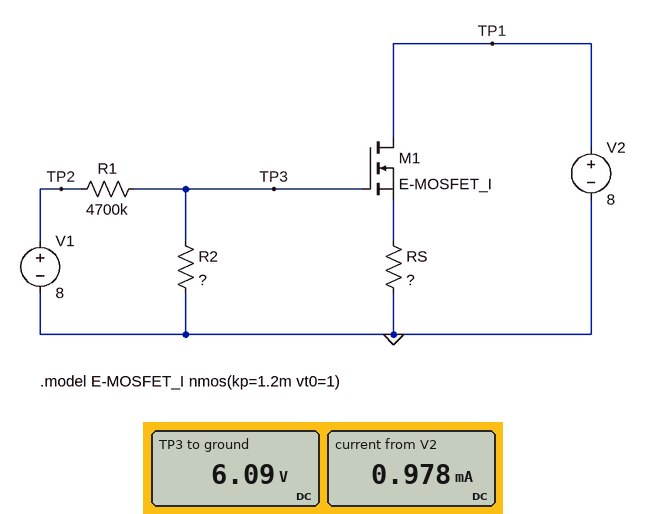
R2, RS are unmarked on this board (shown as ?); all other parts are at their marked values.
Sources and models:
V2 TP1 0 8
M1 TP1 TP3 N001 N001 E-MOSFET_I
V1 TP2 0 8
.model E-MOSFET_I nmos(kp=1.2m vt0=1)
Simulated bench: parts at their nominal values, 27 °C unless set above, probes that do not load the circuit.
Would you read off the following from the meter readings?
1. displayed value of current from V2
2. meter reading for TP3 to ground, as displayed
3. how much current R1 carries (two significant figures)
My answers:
0.978 mA
6.09 V
410 nA
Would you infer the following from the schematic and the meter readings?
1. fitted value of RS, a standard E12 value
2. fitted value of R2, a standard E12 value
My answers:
3.9 kΩ
15 MΩ
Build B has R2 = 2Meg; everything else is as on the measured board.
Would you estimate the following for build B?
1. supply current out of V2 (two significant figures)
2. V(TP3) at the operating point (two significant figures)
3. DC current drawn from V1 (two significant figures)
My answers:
210 µA
2.4 V
1.2 µA
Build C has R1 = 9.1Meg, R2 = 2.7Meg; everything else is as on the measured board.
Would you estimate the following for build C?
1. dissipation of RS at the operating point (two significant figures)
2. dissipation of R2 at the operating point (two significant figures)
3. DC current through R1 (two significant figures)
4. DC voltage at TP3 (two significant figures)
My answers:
43 µW
1.2 µW
680 nA
1.8 V
